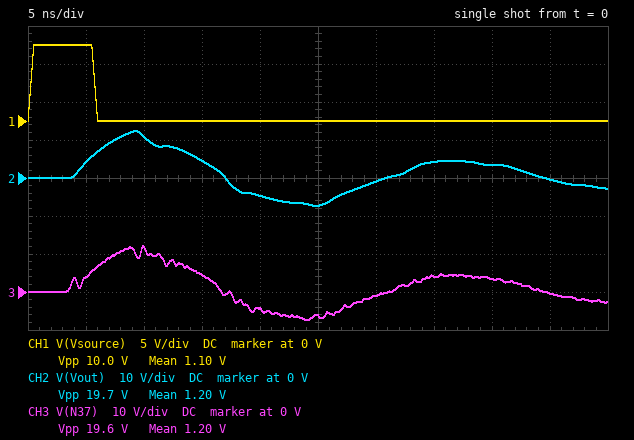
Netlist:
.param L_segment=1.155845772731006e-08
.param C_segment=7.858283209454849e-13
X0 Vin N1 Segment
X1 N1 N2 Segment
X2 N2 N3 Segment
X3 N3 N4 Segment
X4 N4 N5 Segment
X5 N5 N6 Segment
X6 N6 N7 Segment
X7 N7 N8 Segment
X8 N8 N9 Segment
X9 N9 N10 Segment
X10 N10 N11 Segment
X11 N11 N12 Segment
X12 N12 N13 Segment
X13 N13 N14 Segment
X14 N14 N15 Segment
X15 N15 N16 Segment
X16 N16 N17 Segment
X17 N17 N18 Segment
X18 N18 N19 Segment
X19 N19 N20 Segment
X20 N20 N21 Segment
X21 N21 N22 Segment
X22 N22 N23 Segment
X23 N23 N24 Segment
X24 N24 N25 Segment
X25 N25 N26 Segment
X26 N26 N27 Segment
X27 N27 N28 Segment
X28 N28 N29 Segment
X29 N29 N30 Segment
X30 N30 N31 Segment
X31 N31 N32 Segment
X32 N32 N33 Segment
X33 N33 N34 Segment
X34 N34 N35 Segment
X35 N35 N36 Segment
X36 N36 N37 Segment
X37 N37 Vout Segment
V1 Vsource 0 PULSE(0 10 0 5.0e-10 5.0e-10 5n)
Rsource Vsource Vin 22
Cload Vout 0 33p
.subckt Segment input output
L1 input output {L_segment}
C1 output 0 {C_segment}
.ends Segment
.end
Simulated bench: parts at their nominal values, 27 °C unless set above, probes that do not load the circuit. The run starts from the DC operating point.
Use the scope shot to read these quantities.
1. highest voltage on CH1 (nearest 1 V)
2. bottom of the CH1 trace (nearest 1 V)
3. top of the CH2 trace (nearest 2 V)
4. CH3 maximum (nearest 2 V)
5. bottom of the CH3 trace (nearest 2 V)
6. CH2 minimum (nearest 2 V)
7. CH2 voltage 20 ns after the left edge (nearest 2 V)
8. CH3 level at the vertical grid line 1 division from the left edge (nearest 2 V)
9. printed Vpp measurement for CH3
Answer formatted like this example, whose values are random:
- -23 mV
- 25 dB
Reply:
- 10 V
- 0 V
- 12 V
- 12 V
- -8 V
- -8 V
- -4 V
- 4 V
- 19.6 V
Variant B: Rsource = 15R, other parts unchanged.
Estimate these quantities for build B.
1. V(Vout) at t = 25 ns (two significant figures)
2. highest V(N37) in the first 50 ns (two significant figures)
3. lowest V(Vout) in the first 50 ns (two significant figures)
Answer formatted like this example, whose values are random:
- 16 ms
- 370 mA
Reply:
- -9.1 V
- 13 V
- -9.2 V
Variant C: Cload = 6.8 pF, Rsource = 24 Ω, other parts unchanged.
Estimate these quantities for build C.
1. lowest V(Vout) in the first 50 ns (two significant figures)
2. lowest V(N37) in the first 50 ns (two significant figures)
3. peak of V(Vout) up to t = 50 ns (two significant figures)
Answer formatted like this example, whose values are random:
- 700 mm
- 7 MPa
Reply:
- -13 V
- -12 V
- 17 V
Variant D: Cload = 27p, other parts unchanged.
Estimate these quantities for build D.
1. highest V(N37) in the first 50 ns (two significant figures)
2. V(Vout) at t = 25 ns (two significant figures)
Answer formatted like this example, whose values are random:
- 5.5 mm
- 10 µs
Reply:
- 13 V
- -6.7 V
